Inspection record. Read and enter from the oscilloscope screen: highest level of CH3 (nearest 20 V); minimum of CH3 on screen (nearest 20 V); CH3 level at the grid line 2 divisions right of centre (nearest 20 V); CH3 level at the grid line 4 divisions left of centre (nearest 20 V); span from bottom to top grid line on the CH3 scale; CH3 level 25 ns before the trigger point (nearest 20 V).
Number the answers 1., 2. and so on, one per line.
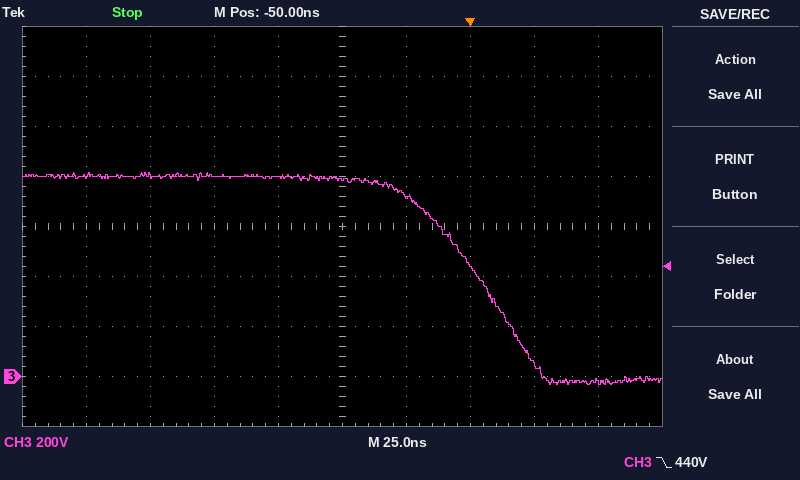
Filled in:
1. 820 V
2. -40 V
3. 440 V
4. 800 V
5. 1.6 kV
6. 720 V
